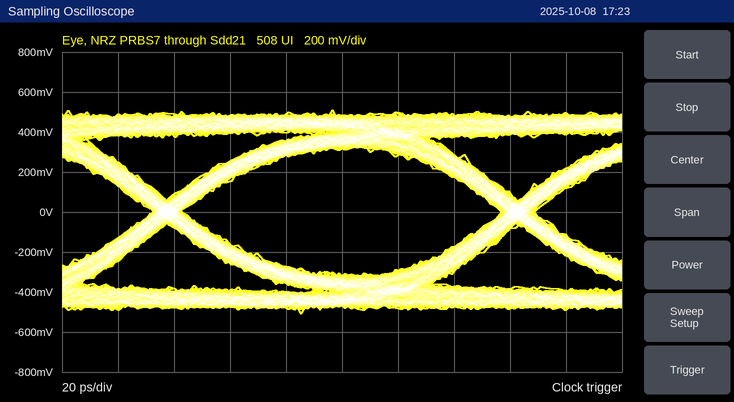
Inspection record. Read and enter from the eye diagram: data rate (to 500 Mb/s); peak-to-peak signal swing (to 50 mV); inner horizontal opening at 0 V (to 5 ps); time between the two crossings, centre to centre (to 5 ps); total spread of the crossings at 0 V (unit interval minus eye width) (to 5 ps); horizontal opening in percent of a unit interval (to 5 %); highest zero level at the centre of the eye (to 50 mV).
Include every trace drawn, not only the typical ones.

8.0 Gb/s
1.00 V
115 ps
125 ps
10 ps
90 %
-300 mV
